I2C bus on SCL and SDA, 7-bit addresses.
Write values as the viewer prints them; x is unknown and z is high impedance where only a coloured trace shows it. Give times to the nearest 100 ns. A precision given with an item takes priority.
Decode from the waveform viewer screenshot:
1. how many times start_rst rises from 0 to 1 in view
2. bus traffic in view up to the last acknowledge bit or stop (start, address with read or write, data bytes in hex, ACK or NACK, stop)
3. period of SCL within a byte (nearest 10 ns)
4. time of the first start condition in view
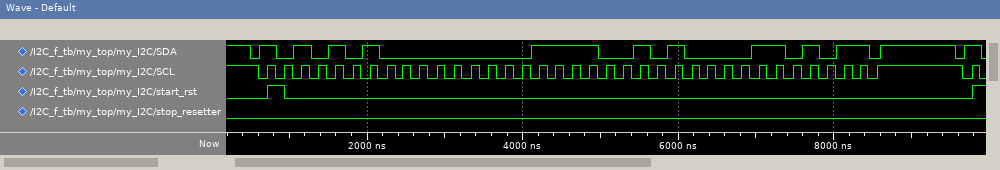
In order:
2
start, address 55 write ACK, 01 NACK, CA ACK, 35 NACK, stop
220 ns
500 ns
